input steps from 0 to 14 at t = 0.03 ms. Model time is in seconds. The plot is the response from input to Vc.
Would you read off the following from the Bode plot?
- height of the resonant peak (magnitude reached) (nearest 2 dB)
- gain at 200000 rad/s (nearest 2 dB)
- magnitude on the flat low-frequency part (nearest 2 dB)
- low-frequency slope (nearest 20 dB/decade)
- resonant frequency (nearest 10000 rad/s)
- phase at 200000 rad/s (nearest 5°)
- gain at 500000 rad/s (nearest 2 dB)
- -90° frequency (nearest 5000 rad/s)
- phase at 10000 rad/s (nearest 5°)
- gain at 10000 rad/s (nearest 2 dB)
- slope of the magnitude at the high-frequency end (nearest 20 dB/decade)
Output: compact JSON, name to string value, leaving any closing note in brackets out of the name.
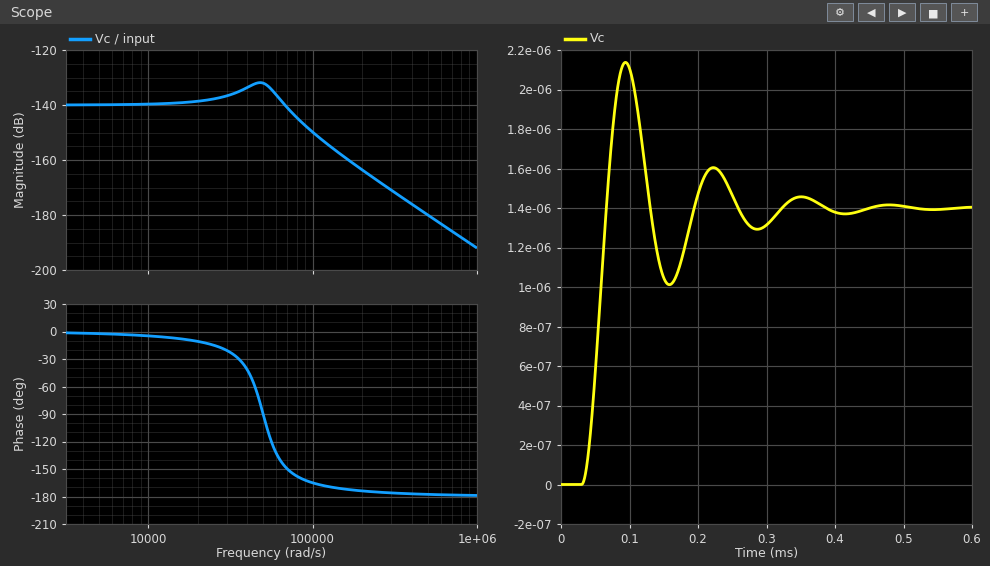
{"height of the resonant peak (magnitude reached)": "-132 dB", "gain at 200000 rad/s": "-164 dB", "magnitude on the flat low-frequency part": "-140 dB", "low-frequency slope": "0 dB/decade", "resonant frequency": "50000 rad/s", "phase at 200000 rad/s": "-175°", "gain at 500000 rad/s": "-180 dB", "-90° frequency": "50000 rad/s", "phase at 10000 rad/s": "-5°", "gain at 10000 rad/s": "-140 dB", "slope of the magnitude at the high-frequency end": "-40 dB/decade"}
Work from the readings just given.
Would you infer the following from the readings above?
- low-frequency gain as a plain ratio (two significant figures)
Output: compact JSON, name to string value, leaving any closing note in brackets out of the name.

{"low-frequency gain as a plain ratio": "0.00000010"}
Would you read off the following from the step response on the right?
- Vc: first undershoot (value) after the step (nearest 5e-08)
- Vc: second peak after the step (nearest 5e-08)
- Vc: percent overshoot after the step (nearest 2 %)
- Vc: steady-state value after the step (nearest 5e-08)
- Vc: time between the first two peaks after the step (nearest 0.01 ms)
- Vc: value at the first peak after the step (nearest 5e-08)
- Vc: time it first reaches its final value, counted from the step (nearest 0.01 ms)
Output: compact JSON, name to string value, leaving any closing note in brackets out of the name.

{"Vc: first undershoot (value) after the step": "0.00000100", "Vc: second peak after the step": "0.00000160", "Vc: percent overshoot after the step": "52 %", "Vc: steady-state value after the step": "0.00000140", "Vc: time between the first two peaks after the step": "0.13 ms", "Vc: value at the first peak after the step": "0.00000215", "Vc: time it first reaches its final value, counted from the step": "0.04 ms"}
